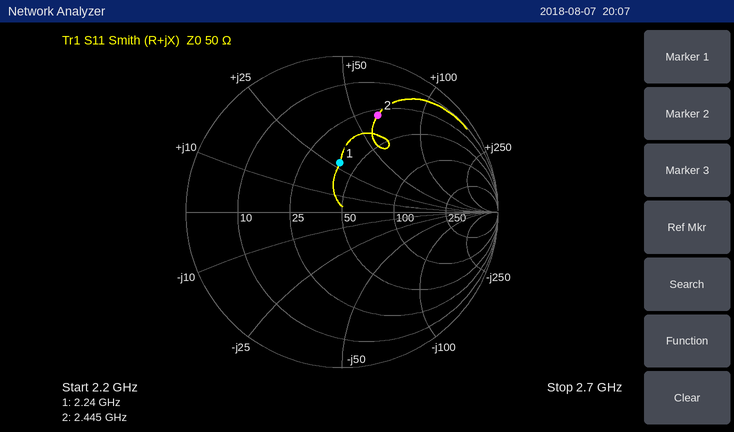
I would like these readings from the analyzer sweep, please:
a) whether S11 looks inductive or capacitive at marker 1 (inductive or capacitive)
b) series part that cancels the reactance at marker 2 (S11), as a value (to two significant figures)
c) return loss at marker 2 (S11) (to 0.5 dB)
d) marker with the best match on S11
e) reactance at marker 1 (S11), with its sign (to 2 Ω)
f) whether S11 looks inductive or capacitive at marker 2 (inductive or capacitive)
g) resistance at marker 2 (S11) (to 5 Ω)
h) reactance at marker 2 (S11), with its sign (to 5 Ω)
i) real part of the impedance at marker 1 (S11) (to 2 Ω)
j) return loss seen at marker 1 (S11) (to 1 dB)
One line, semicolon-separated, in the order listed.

inductive; 1.0 pF; 3.5 dB; marker 1; +28 Ω; inductive; 30 Ω; +65 Ω; 40 Ω; 10 dB
